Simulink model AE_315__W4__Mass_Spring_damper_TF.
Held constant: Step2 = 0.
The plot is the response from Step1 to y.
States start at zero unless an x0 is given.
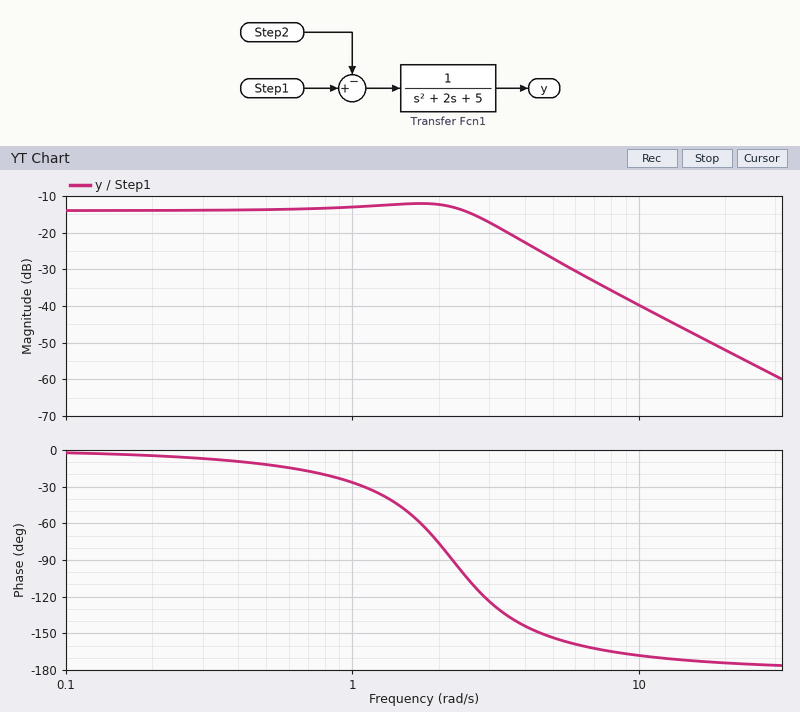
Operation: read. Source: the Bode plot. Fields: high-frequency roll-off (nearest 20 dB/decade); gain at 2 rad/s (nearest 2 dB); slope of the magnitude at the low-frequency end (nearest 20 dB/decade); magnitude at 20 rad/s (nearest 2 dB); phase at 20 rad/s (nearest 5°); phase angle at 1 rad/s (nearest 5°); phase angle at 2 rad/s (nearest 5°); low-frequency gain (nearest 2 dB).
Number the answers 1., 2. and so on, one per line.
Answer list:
1. -40 dB/decade
2. -12 dB
3. 0 dB/decade
4. -52 dB
5. -175°
6. -25°
7. -75°
8. -14 dB
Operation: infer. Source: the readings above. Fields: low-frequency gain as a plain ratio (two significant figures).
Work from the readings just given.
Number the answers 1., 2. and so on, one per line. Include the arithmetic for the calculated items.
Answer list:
1. 10^(-14 / 20) = 0.20
